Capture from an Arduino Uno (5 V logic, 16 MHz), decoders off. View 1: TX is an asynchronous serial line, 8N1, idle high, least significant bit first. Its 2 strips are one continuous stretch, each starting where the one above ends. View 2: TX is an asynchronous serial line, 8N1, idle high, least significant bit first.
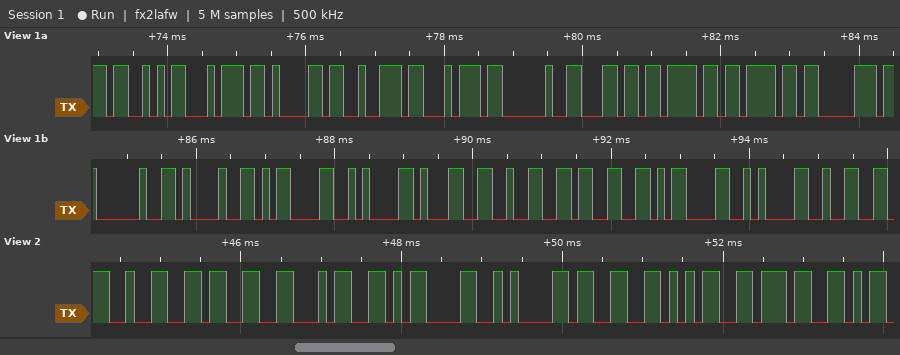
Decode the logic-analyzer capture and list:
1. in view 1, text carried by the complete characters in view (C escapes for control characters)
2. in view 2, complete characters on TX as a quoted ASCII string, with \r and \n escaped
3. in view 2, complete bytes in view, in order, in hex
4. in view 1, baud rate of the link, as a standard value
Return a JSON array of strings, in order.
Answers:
["\"Start loop !\\r\\n123\\r\\n2\"", "\"234\\r\\n357\"", "0x32 0x33 0x34 0x0D 0x0A 0x33 0x35 0x37", "9600 baud"]
